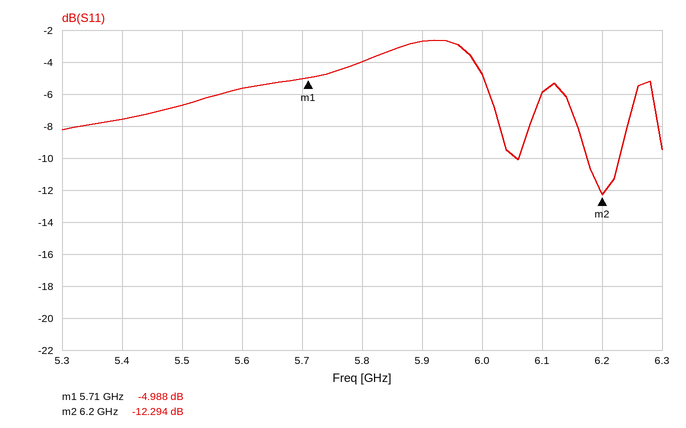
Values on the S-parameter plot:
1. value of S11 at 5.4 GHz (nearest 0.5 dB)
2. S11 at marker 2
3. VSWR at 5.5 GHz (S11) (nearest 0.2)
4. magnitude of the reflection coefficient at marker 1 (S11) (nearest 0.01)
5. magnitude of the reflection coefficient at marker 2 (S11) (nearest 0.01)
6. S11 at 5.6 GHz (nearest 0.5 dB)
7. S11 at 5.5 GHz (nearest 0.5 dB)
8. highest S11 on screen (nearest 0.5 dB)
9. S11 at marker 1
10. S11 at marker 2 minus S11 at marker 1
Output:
-7.5 dB
-12.294 dB
2.8
0.56
0.24
-5.5 dB
-6.5 dB
-2.5 dB
-4.988 dB
-7.306 dB
